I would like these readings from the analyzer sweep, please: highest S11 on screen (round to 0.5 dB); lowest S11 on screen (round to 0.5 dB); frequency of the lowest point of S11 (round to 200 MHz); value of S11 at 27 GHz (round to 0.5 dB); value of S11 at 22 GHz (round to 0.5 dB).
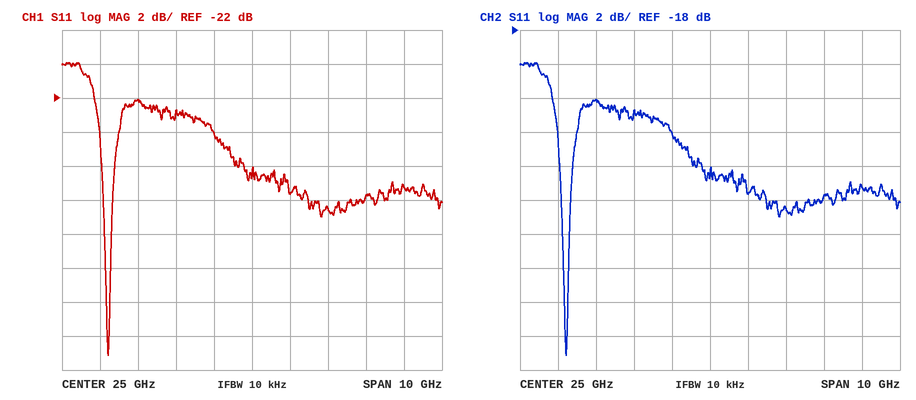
-20.0 dB
-37.0 dB
21.2 GHz
-28.5 dB
-22.0 dB
